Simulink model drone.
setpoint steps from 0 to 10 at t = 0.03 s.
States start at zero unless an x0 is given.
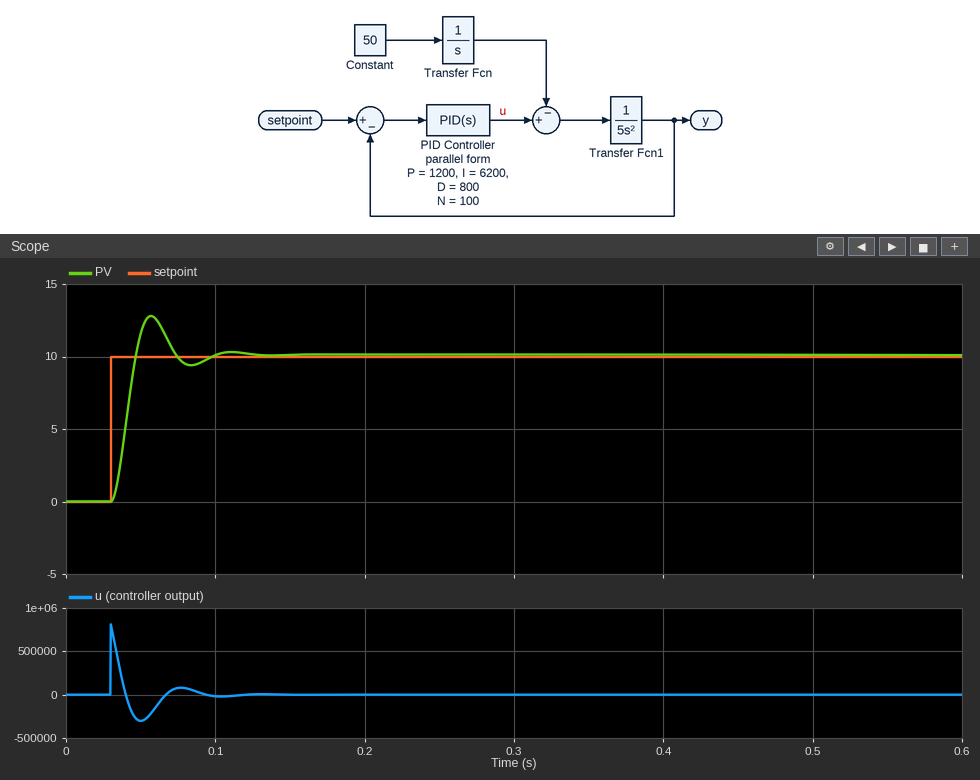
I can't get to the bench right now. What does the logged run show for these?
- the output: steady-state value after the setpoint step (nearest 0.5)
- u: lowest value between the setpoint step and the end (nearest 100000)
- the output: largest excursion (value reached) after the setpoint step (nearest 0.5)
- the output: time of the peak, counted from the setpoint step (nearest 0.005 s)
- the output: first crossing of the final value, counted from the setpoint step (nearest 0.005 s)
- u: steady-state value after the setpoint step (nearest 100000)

10.0
-300000
13.0
0.025 s
0.015 s
0
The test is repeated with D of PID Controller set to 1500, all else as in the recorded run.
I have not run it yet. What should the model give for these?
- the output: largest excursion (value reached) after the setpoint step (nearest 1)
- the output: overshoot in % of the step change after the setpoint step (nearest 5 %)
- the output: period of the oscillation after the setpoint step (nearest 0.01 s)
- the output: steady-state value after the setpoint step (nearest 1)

14
40 %
0.04 s
10
